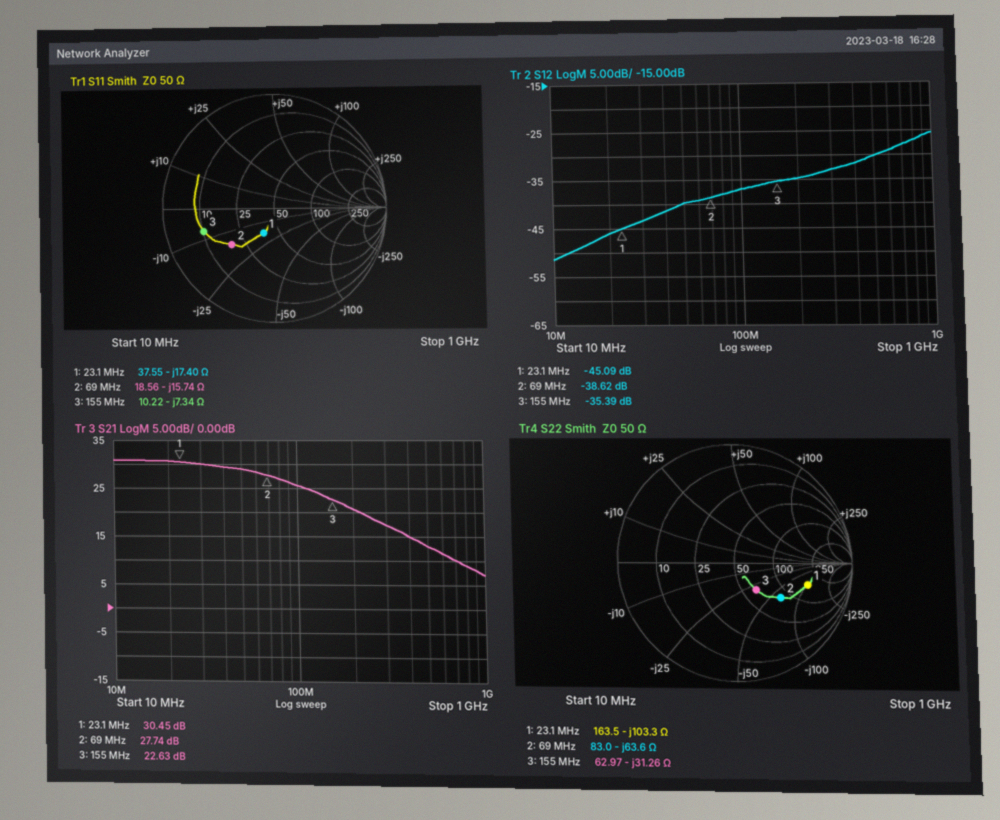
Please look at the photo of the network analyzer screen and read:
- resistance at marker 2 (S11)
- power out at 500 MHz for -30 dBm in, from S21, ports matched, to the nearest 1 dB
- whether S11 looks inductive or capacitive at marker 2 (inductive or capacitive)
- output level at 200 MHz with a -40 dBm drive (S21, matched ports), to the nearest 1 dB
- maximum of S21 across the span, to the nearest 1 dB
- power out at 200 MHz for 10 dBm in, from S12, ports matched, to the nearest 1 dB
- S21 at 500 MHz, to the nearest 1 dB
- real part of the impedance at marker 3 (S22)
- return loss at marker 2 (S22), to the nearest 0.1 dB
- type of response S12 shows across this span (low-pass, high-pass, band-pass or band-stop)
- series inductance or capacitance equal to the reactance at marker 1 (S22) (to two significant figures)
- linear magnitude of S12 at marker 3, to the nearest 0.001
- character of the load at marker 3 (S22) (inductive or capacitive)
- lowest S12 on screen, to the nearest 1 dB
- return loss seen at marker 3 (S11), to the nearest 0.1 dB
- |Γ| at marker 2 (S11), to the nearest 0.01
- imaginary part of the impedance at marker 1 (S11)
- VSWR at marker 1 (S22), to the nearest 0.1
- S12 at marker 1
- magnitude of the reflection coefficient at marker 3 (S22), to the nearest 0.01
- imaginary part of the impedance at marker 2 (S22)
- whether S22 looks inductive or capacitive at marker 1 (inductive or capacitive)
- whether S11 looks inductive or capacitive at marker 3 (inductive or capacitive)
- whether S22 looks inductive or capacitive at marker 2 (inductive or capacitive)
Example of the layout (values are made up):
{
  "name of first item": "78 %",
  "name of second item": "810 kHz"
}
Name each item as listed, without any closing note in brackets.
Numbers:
{
  "resistance at marker 2": "18.56 Ω",
  "power out at 500 MHz for -30 dBm in, from S21, ports matched, to the nearest 1 dB": "-17 dBm",
  "whether S11 looks inductive or capacitive at marker 2": "capacitive",
  "output level at 200 MHz with a -40 dBm drive (S21, matched ports), to the nearest 1 dB": "-19 dBm",
  "maximum of S21 across the span, to the nearest 1 dB": "31 dB",
  "power out at 200 MHz for 10 dBm in, from S12, ports matched, to the nearest 1 dB": "-25 dBm",
  "S21 at 500 MHz, to the nearest 1 dB": "13 dB",
  "real part of the impedance at marker 3": "62.97 Ω",
  "return loss at marker 2 (S22), to the nearest 0.1 dB": "6.3 dB",
  "type of response S12 shows across this span": "high-pass",
  "series inductance or capacitance equal to the reactance at marker 1 (S22)": "67 pF",
  "linear magnitude of S12 at marker 3, to the nearest 0.001": "0.017",
  "character of the load at marker 3 (S22)": "capacitive",
  "lowest S12 on screen, to the nearest 1 dB": "-51 dB",
  "return loss seen at marker 3 (S11), to the nearest 0.1 dB": "3.5 dB",
  "|Γ| at marker 2 (S11), to the nearest 0.01": "0.50",
  "imaginary part of the impedance at marker 1": "-17.40 Ω",
  "VSWR at marker 1 (S22), to the nearest 0.1": "4.7",
  "S12 at marker 1": "-45.09 dB",
  "magnitude of the reflection coefficient at marker 3 (S22), to the nearest 0.01": "0.29",
  "imaginary part of the impedance at marker 2": "-63.6 Ω",
  "whether S22 looks inductive or capacitive at marker 1": "capacitive",
  "whether S11 looks inductive or capacitive at marker 3": "capacitive",
  "whether S22 looks inductive or capacitive at marker 2": "capacitive"
}
